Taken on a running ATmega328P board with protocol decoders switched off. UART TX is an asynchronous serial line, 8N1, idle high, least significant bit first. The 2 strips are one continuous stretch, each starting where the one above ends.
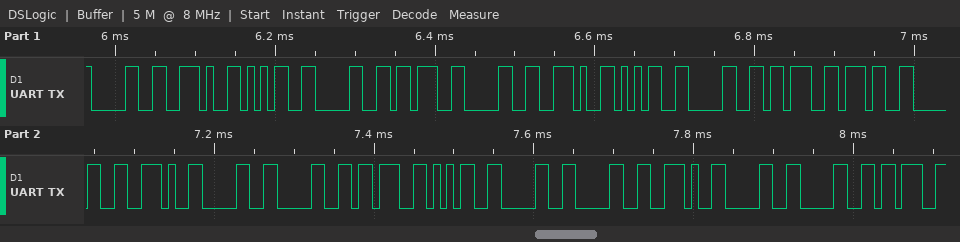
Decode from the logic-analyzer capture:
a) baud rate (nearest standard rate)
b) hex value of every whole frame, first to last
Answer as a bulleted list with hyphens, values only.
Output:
- 115200 baud
- 30 2E 35 30 3B 30 2E 35 30 3B 37 30 2E 30 30 3B 35 30 30 2E 30 30 3B
